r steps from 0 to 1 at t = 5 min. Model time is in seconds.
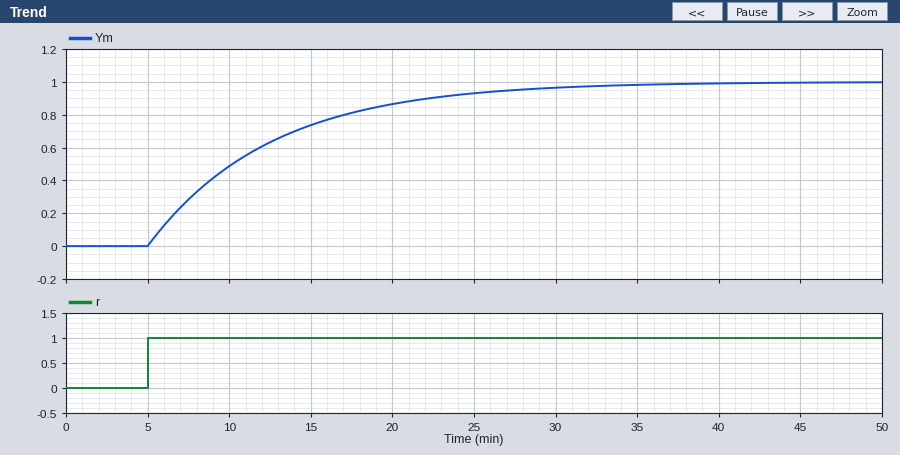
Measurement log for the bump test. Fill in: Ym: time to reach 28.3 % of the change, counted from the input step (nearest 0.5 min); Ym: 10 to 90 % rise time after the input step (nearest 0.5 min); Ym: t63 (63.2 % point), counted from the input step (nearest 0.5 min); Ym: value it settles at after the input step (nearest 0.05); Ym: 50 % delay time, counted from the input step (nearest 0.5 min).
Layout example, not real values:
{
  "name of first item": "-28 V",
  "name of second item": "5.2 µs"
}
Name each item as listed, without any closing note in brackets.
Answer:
{
  "Ym: time to reach 28.3 % of the change, counted from the input step": "2.5 min",
  "Ym: 10 to 90 % rise time after the input step": "16.5 min",
  "Ym: t63 (63.2 % point), counted from the input step": "7.5 min",
  "Ym: value it settles at after the input step": "1.00",
  "Ym: 50 % delay time, counted from the input step": "5.0 min"
}
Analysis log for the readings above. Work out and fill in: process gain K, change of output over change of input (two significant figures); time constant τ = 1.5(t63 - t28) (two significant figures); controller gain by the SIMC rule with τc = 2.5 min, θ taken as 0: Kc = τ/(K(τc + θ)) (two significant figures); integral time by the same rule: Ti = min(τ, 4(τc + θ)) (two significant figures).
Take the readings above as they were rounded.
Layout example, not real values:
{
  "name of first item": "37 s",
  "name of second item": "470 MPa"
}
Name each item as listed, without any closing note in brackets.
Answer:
{
  "process gain K, change of output over change of input": "1.0",
  "time constant τ = 1.5(t63 - t28)": "7.5 min",
  "controller gain by the SIMC rule with τc = 2.5 min, θ taken as 0: Kc = τ/(K(τc + θ))": "3.0",
  "integral time by the same rule: Ti = min(τ, 4(τc + θ))": "7.5 min"
}
